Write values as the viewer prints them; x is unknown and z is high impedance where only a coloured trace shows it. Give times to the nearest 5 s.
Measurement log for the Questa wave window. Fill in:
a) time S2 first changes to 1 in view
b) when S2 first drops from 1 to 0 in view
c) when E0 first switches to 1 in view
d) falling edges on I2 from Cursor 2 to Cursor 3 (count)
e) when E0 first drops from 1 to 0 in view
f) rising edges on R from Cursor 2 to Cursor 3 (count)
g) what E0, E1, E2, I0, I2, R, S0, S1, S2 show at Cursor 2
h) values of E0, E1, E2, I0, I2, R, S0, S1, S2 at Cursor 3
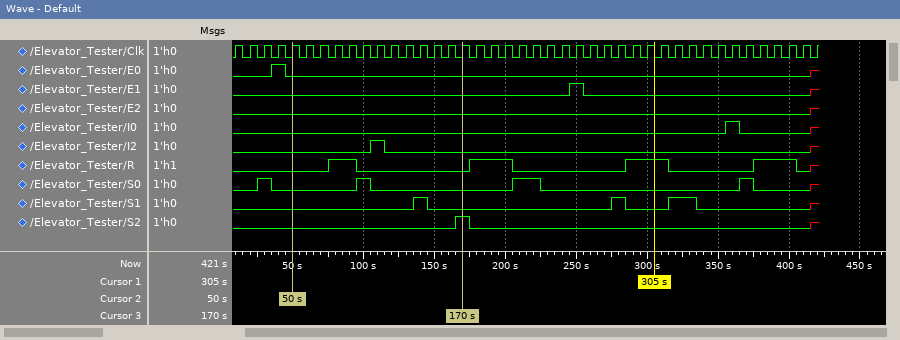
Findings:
165 s
175 s
35 s
1
45 s
1
E0=0, E1=0, E2=0, I0=0, I2=0, R=0, S0=0, S1=0, S2=0
E0=0, E1=0, E2=0, I0=0, I2=0, R=0, S0=0, S1=0, S2=1
